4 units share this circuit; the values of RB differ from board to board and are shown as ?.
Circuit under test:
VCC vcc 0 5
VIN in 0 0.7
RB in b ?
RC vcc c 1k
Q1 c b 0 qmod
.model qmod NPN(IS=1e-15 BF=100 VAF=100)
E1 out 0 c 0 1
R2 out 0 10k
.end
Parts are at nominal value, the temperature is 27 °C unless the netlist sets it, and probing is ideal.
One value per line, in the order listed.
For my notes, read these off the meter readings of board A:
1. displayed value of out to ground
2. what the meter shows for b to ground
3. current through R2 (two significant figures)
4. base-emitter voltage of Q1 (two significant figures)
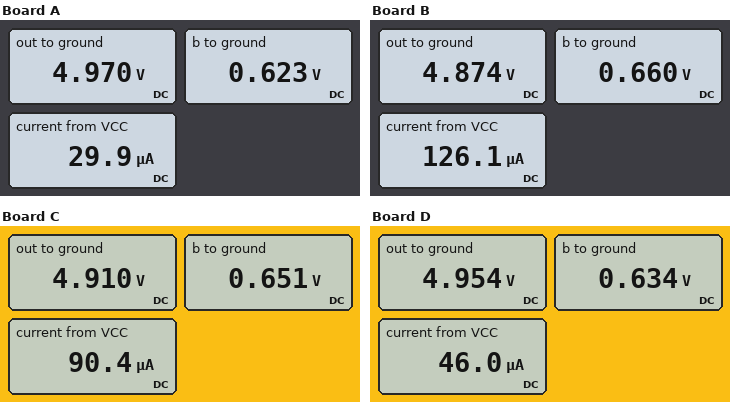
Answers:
4.970 V
0.623 V
500 µA
620 mV
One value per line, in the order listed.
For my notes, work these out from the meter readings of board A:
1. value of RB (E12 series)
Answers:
270 kΩ
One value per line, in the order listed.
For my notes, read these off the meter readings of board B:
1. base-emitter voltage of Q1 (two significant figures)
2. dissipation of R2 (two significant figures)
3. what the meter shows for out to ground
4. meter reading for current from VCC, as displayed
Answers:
660 mV
2.4 mW
4.874 V
126.1 µA
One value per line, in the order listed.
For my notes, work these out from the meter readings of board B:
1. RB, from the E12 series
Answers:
33 kΩ
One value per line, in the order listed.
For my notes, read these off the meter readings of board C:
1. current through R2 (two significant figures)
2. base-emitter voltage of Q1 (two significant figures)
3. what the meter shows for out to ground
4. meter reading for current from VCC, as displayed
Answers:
490 µA
650 mV
4.910 V
90.4 µA
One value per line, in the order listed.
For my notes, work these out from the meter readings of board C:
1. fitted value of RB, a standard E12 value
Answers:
56 kΩ
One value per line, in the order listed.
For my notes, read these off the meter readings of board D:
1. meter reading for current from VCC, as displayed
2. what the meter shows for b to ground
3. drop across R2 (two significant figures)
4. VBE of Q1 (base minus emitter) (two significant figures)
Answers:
46.0 µA
0.634 V
5.0 V
630 mV
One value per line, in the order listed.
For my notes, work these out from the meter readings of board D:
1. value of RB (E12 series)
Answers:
150 kΩ
